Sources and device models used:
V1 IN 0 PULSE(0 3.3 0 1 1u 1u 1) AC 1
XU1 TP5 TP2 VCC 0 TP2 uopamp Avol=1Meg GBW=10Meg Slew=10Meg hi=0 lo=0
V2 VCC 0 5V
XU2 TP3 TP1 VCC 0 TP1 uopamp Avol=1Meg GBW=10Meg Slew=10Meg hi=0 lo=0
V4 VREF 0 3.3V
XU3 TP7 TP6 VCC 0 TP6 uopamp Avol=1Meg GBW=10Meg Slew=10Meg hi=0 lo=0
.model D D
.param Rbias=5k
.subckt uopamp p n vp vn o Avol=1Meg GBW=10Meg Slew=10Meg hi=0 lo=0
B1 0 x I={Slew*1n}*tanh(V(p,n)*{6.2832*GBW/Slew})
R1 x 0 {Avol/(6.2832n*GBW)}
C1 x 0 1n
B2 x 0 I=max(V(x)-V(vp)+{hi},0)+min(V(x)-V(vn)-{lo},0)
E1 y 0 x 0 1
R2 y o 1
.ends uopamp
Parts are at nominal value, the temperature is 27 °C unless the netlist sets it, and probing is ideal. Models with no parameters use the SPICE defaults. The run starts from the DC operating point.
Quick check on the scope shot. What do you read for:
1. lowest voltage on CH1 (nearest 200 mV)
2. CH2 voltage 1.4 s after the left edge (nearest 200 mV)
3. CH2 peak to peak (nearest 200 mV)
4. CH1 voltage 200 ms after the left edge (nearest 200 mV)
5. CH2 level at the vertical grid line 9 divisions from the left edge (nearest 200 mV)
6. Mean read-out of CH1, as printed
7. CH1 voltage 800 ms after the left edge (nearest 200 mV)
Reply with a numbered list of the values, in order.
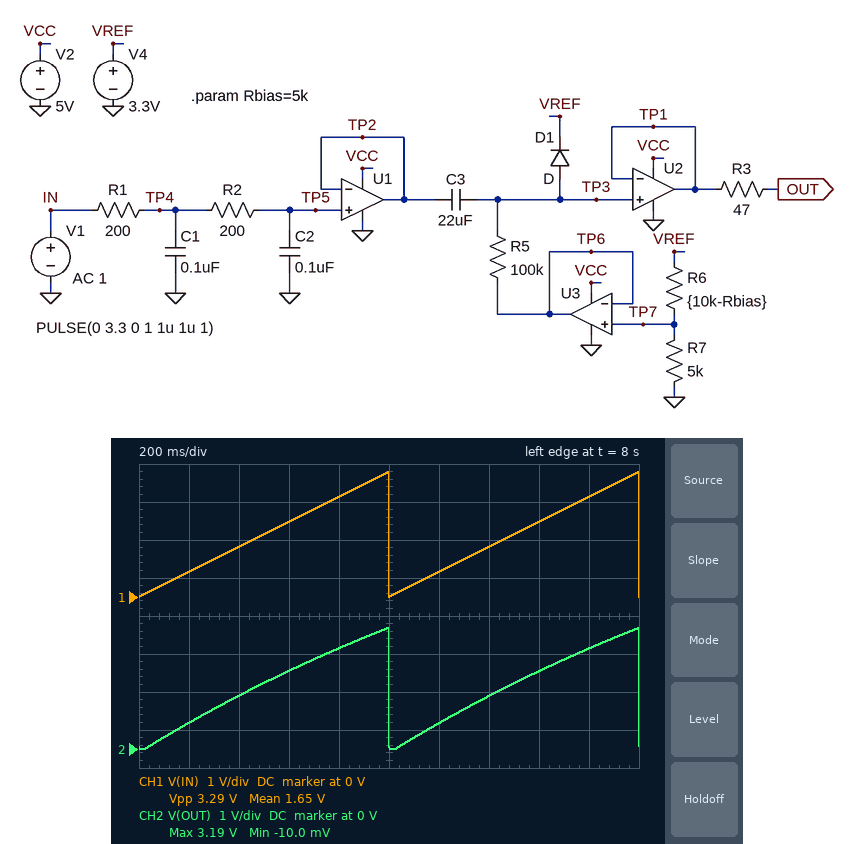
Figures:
1. 0 V
2. 1.4 V
3. 3.2 V
4. 600 mV
5. 2.6 V
6. 1.65 V
7. 2.6 V
